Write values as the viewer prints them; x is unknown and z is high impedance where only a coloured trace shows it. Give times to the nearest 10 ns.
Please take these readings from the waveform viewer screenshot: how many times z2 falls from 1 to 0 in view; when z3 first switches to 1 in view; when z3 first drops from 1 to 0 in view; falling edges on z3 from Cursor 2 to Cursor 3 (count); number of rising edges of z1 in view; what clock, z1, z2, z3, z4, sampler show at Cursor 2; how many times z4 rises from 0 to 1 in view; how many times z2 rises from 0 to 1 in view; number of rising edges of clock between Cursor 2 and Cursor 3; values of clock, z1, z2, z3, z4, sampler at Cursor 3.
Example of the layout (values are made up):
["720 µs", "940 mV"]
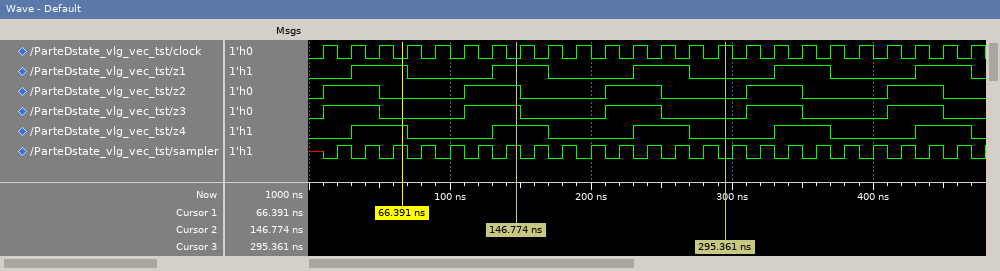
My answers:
["5", "10 ns", "50 ns", "2", "5", "clock=0, z1=1, z2=1, z3=1, z4=1, sampler=1", "5", "5", "8", "clock=1, z1=0, z2=0, z3=0, z4=0, sampler=0"]
